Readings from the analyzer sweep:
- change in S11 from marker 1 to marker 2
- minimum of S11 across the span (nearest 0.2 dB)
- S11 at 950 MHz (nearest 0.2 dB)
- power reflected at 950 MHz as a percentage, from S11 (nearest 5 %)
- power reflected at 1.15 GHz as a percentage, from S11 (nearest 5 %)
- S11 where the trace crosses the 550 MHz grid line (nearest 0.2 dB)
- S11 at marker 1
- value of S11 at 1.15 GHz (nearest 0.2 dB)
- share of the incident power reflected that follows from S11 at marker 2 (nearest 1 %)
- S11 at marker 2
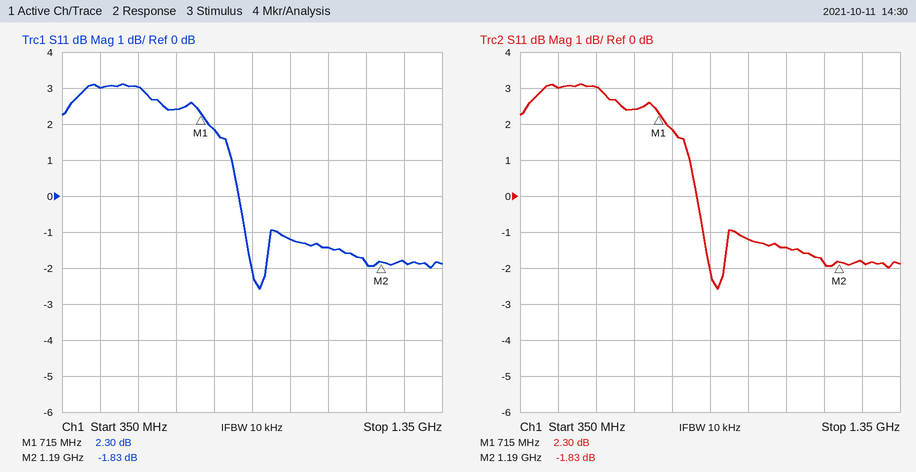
-4.13 dB
-2.6 dB
-1.2 dB
75 %
65 %
3.0 dB
2.30 dB
-1.8 dB
66 %
-1.83 dB
